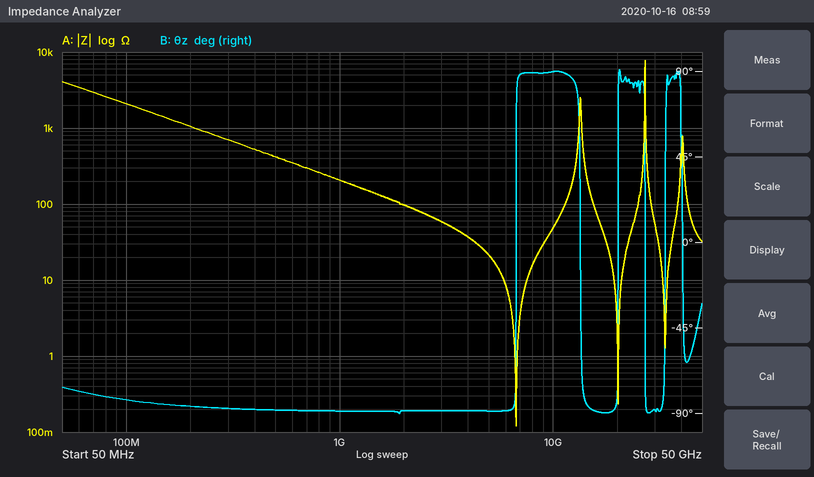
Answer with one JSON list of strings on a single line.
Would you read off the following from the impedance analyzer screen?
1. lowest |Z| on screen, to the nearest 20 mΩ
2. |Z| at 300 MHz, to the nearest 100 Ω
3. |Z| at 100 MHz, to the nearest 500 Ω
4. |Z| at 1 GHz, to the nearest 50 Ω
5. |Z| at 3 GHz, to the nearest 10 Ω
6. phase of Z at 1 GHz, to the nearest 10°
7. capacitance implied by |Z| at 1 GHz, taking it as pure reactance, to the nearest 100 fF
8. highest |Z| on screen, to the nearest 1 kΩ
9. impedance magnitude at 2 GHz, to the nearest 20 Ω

["120 mΩ", "700 Ω", "2.0 kΩ", "200 Ω", "60 Ω", "-90°", "800 fF", "8 kΩ", "100 Ω"]
